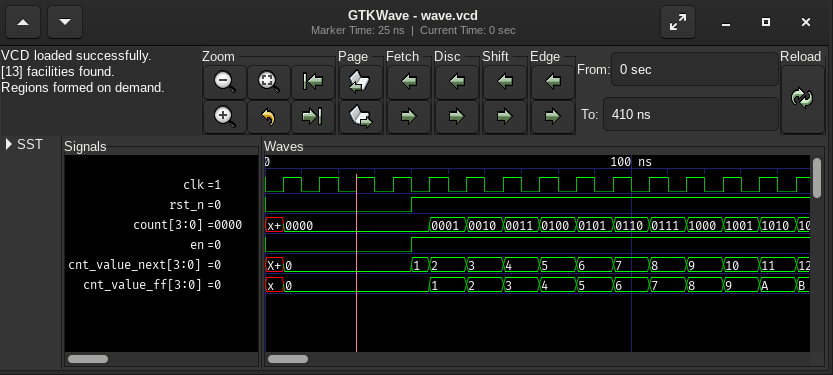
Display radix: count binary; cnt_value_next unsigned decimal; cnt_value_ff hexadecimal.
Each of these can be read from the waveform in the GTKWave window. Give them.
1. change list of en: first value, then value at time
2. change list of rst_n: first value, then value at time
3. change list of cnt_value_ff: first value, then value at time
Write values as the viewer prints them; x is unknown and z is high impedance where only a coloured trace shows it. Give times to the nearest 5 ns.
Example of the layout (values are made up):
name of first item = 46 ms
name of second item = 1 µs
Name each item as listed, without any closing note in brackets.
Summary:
change list of en: first value, then value at time = 0, 1 at 40 ns
change list of rst_n: first value, then value at time = 0, 1 at 40 ns
change list of cnt_value_ff: first value, then value at time = x, 0 at 5 ns, 1 at 45 ns, 2 at 55 ns, 3 at 65 ns, 4 at 75 ns, 5 at 85 ns, 6 at 95 ns, 7 at 105 ns, 8 at 115 ns, 9 at 125 ns, A at 135 ns, B at 145 ns
